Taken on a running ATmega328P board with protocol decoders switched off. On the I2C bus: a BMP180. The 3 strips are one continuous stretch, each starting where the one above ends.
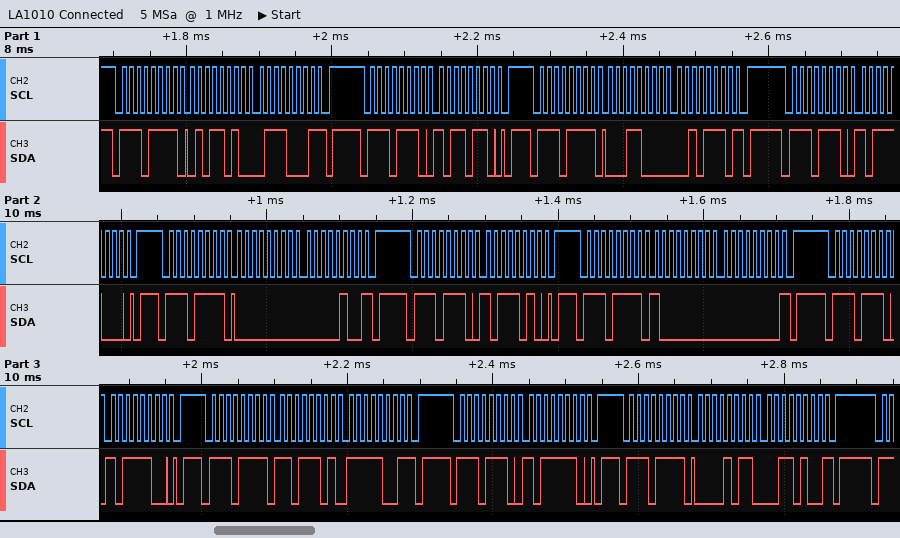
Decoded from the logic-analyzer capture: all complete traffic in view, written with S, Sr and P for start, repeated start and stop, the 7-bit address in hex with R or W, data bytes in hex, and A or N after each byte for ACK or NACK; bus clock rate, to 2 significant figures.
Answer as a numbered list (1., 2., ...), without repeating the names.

1. S 77R A 5A A 71 N P S 77W A B6 A P S 77R A 18 A 2E N P S 77W A B8 A P S 77R A 00 A 04 N P S 77W A BA A P S 77R A 80 A 00 N P S 77W A BC A P S 77R A DD A F9 N P S 77W A BE A P S 77R A 0B A 34 N P
2. 100 kHz
